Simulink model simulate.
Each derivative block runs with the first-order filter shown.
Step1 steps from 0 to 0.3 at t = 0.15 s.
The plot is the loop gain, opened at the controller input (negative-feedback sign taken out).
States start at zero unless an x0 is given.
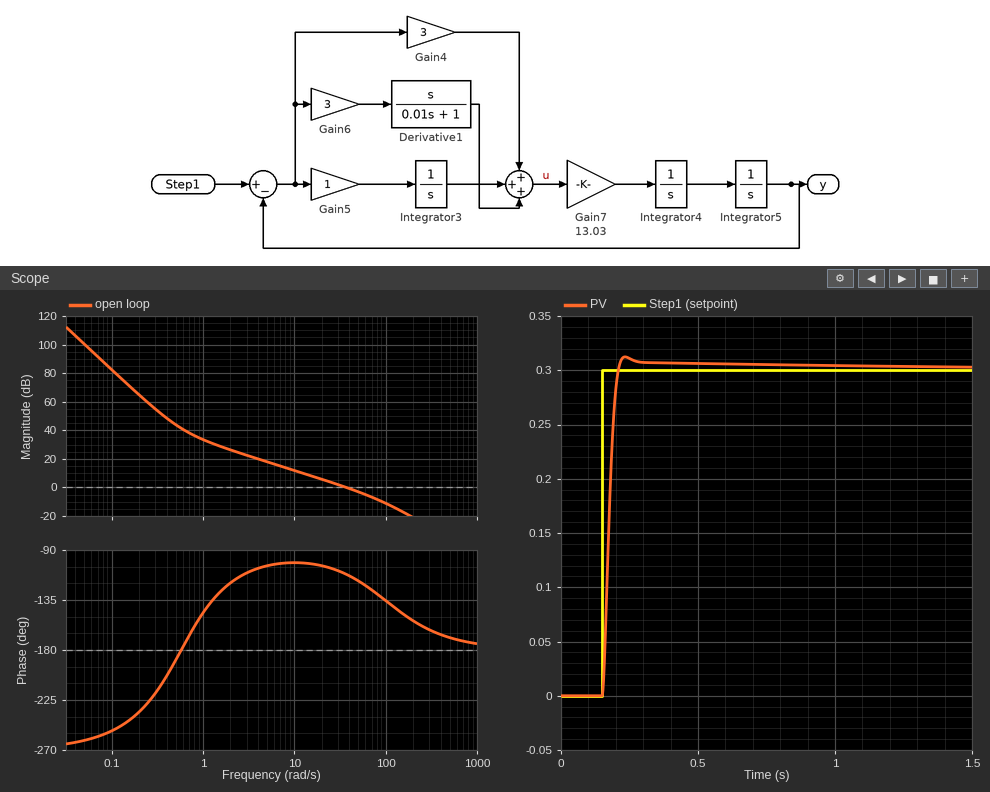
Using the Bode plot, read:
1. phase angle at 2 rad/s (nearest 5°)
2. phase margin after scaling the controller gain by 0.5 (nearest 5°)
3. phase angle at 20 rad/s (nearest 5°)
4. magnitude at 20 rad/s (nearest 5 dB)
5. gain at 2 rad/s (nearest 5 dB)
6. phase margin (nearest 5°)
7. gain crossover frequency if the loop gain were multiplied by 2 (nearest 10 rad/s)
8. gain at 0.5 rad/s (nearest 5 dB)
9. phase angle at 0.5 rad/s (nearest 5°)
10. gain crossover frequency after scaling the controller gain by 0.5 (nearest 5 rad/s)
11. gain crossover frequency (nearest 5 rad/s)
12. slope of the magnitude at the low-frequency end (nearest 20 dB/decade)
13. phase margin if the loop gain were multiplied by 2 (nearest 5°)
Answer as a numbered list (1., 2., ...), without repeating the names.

1. -120°
2. 75°
3. -105°
4. 5 dB
5. 25 dB
6. 70°
7. 70 rad/s
8. 45 dB
9. -190°
10. 20 rad/s
11. 35 rad/s
12. -60 dB/decade
13. 55°
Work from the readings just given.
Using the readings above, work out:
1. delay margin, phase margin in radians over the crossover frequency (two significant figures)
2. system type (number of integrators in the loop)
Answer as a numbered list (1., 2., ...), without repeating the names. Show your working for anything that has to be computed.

1. 70 × π / 180 / 35 = 0.035 s
2. 3
